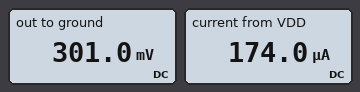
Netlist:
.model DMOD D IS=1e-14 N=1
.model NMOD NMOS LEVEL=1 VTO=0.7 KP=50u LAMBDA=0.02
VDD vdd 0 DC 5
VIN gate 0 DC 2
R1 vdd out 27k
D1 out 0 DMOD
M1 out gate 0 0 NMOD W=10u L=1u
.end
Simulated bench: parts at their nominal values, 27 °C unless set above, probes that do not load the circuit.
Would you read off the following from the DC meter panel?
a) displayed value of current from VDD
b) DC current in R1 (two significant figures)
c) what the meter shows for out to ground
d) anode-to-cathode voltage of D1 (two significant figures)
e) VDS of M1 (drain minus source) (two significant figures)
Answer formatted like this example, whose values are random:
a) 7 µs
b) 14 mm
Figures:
a) 174.0 µA
b) 170 µA
c) 301.0 mV
d) 300 mV
e) 300 mV
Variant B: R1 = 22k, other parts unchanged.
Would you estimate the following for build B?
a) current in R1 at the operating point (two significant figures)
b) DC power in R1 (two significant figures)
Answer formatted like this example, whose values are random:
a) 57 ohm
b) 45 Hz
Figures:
a) 210 µA
b) 970 µW
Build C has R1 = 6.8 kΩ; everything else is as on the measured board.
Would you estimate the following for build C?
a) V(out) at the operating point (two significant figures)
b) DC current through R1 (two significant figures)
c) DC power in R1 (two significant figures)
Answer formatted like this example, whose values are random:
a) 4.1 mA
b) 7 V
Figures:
a) 630 mV
b) 640 µA
c) 2.8 mW
